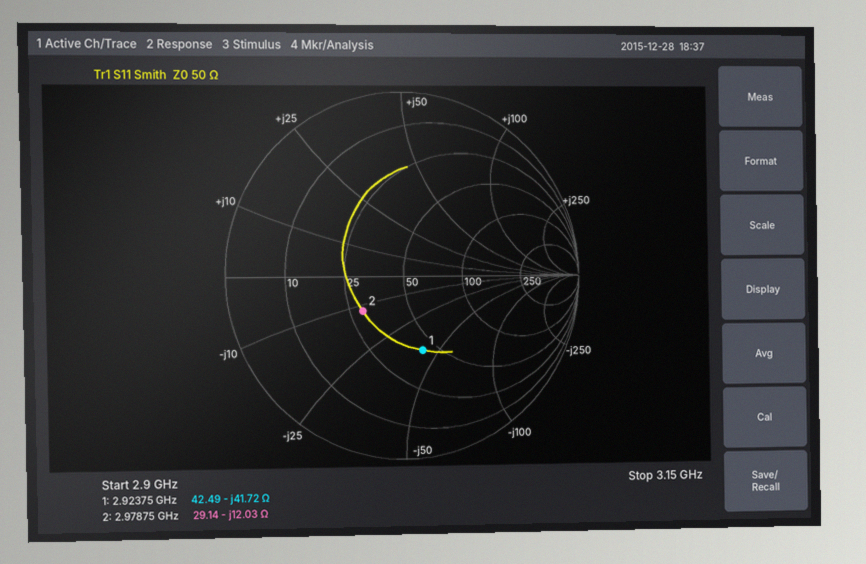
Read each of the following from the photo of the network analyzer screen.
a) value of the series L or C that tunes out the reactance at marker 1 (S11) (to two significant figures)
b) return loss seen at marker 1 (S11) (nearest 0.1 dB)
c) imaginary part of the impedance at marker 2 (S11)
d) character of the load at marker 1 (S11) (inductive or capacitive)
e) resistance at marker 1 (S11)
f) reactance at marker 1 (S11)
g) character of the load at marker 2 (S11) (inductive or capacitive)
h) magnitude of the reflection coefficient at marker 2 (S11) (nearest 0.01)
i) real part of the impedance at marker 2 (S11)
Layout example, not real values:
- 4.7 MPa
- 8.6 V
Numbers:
- 2.3 nH
- 7.6 dB
- -12.03 Ω
- capacitive
- 42.49 Ω
- -41.72 Ω
- capacitive
- 0.30
- 29.14 Ω
